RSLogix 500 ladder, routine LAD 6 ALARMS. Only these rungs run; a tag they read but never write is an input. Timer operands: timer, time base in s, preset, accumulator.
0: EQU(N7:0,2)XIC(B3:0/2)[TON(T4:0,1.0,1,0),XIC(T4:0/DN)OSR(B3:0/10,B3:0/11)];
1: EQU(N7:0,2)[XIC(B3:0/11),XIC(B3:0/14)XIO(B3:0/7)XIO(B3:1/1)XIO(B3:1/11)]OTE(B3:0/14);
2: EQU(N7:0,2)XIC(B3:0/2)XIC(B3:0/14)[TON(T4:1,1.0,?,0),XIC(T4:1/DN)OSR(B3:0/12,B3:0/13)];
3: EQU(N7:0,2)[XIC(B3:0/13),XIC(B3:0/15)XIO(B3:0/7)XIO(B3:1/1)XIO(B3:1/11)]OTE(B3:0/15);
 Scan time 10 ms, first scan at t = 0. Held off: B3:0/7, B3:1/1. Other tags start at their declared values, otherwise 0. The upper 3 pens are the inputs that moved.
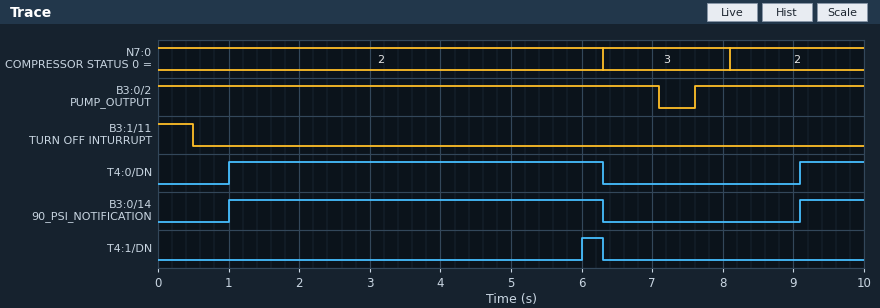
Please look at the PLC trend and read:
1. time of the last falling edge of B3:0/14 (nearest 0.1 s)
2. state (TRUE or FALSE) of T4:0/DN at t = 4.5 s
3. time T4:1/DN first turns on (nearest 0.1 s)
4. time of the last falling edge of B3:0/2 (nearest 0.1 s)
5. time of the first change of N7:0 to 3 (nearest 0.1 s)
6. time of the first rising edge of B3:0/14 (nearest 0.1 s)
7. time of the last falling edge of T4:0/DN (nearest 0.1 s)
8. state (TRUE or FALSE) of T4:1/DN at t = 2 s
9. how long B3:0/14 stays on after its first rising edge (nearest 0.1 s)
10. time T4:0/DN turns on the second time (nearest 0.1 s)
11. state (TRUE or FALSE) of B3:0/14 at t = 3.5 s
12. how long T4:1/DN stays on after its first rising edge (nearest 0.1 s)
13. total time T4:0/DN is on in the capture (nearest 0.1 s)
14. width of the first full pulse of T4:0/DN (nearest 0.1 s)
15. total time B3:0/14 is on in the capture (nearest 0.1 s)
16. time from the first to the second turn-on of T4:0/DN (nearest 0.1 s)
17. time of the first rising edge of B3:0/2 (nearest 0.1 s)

6.3 s
TRUE
6.0 s
7.1 s
6.3 s
1.0 s
6.3 s
FALSE
5.3 s
9.1 s
TRUE
0.3 s
6.2 s
5.3 s
6.2 s
8.1 s
7.6 s
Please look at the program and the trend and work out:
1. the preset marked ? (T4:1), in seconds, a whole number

5 s
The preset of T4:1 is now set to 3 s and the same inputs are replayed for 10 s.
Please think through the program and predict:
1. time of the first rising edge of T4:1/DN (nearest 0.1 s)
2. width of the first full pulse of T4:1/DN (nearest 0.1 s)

4.0 s
2.3 s
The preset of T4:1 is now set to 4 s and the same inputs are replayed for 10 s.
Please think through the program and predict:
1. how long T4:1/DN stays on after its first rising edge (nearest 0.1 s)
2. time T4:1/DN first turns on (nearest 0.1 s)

1.3 s
5.0 s
